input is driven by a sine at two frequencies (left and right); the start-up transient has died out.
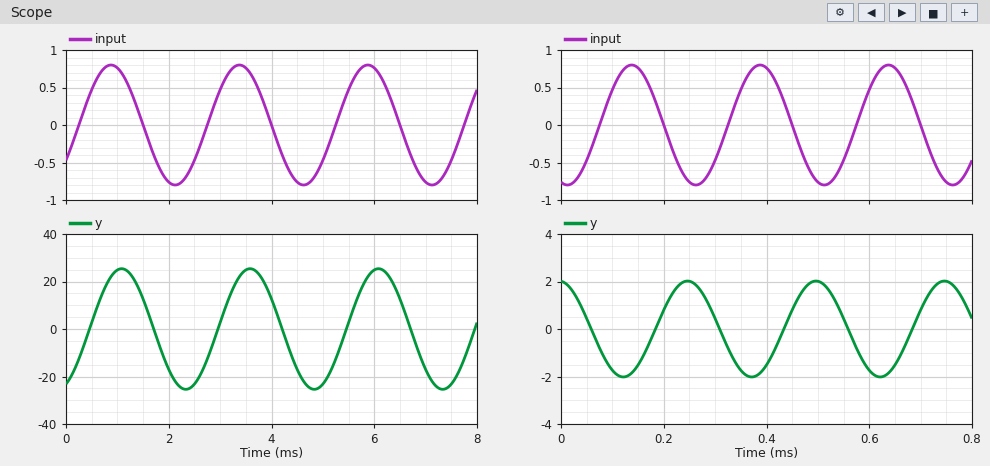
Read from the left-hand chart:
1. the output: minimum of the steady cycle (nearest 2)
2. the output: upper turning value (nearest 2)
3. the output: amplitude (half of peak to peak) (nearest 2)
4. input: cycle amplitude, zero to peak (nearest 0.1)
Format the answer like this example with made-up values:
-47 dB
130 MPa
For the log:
-26
26
26
0.8
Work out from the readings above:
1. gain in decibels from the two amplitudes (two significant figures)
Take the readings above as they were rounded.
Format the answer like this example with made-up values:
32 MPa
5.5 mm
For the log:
30 dB
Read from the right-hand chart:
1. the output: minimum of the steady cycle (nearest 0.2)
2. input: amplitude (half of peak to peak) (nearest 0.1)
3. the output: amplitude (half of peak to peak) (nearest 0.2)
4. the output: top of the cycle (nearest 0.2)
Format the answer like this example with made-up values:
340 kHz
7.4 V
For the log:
-2.0
0.8
2.0
2.0
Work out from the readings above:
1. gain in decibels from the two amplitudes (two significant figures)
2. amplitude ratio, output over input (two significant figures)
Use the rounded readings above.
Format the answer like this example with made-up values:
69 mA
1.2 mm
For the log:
8.0 dB
2.5
